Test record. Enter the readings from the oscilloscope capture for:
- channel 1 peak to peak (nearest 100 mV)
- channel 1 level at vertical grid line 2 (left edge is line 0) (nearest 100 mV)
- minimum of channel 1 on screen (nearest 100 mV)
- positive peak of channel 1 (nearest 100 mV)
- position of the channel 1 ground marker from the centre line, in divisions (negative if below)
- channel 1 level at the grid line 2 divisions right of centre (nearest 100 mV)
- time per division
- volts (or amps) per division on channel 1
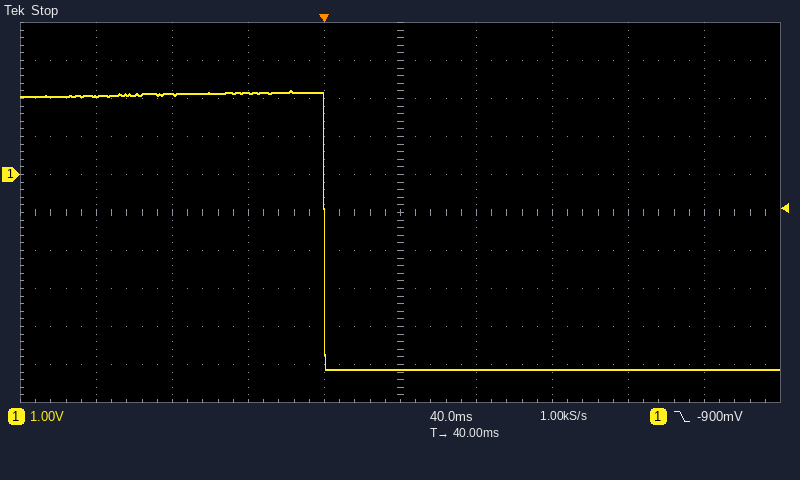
7.3 V
2.1 V
-5.1 V
2.2 V
+1.0 div
-5.1 V
40 ms
1 V
